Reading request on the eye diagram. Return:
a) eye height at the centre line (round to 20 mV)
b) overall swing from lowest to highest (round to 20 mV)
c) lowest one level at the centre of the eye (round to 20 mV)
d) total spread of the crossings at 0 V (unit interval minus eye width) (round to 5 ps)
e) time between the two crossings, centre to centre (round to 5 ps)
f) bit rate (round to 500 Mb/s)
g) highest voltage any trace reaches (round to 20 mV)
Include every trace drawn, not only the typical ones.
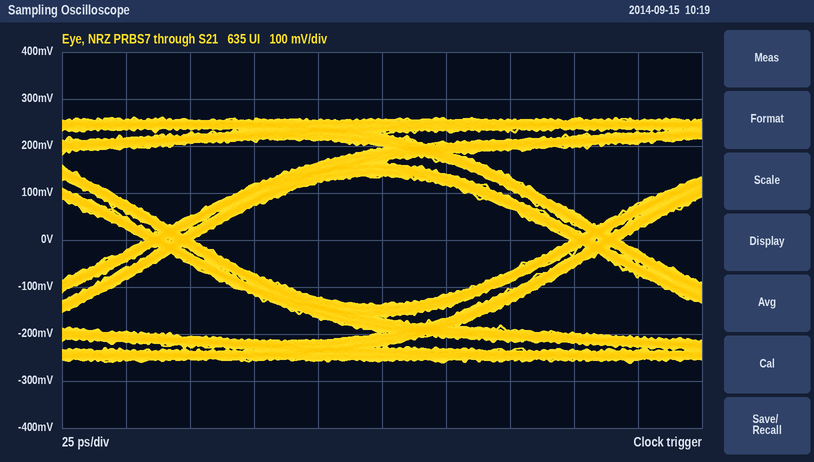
280 mV
520 mV
140 mV
20 ps
165 ps
6.0 Gb/s
260 mV
